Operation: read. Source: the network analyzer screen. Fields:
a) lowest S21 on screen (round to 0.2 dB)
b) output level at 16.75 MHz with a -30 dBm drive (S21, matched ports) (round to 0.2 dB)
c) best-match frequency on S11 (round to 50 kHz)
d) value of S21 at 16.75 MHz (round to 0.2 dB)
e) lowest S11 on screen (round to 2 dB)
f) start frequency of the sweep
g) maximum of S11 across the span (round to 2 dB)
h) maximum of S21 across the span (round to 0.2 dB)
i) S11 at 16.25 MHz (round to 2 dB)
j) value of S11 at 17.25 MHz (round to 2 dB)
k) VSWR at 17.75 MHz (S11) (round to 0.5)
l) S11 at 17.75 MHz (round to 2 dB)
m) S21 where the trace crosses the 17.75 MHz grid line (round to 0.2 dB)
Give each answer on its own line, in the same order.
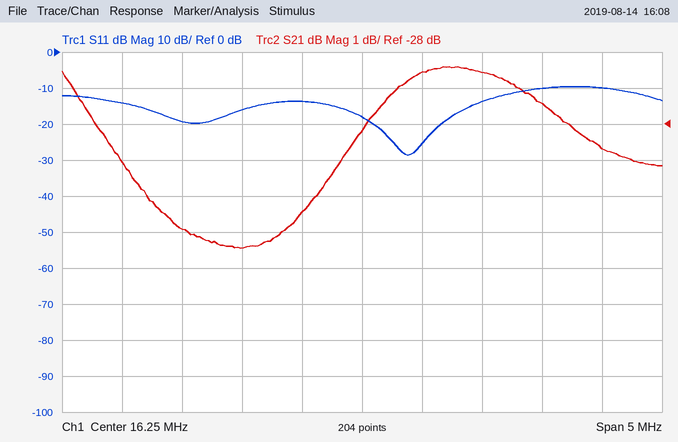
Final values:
-31.4 dB
-56.6 dBm
16.65 MHz
-26.6 dB
-28 dB
13.75 MHz
-10 dB
-26.4 dB
-18 dB
-14 dB
2.0
-10 dB
-27.4 dB
